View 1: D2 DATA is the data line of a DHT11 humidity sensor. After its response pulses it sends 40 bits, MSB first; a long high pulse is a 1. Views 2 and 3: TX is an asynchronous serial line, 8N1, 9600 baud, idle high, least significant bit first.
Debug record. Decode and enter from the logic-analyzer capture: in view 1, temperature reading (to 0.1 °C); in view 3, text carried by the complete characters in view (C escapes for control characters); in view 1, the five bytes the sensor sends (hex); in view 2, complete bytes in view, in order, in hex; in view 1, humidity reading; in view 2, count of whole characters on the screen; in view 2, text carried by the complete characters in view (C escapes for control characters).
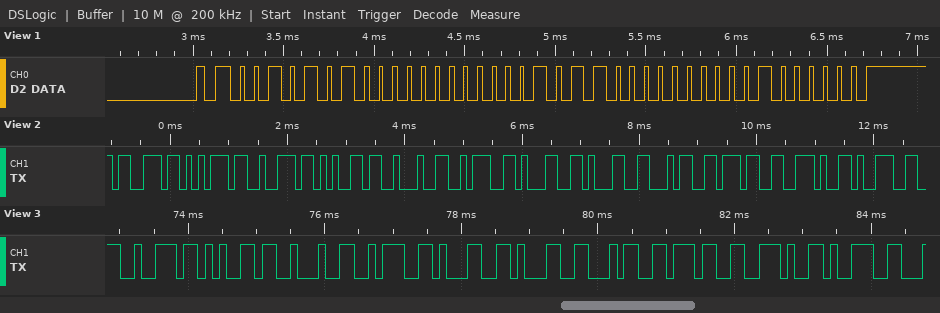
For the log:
22.0 °C
"re\":1147.9"
2A 00 16 00 40
0x73 0x75 0x72 0x65 0x22 0x3A 0x31 0x31 0x34 0x37 0x2E 0x39
42 %
12
"sure\":1147.9"
